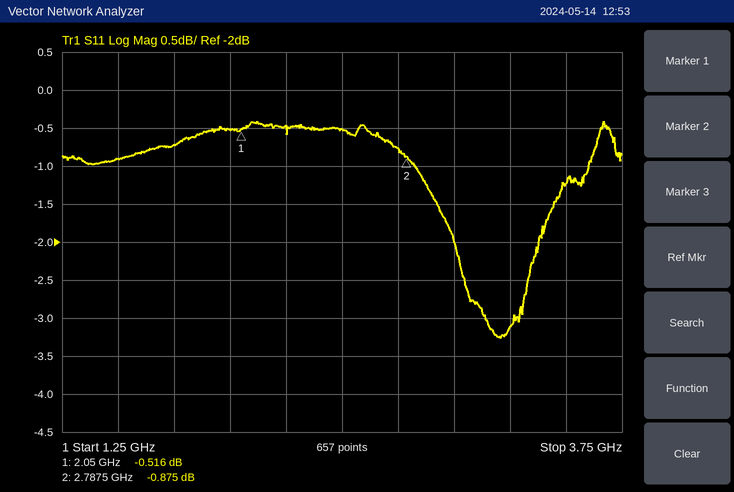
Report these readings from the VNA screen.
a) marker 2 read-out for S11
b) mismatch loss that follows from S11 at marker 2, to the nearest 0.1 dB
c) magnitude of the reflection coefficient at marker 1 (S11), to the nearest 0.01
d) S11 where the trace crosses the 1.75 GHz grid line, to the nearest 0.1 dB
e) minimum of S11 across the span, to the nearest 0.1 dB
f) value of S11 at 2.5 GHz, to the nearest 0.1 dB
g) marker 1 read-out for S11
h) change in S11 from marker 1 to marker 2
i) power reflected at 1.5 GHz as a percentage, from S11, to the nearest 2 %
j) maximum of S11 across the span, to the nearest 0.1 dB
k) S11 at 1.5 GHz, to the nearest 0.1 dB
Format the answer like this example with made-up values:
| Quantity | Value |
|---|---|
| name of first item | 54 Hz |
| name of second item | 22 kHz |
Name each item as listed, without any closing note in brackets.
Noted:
| Quantity | Value |
|---|---|
| marker 2 read-out for S11 | -0.875 dB |
| mismatch loss that follows from S11 at marker 2, to the nearest 0.1 dB | 7.4 dB |
| magnitude of the reflection coefficient at marker 1 (S11), to the nearest 0.01 | 0.94 |
| S11 where the trace crosses the 1.75 GHz grid line, to the nearest 0.1 dB | -0.7 dB |
| minimum of S11 across the span, to the nearest 0.1 dB | -3.3 dB |
| value of S11 at 2.5 GHz, to the nearest 0.1 dB | -0.5 dB |
| marker 1 read-out for S11 | -0.516 dB |
| change in S11 from marker 1 to marker 2 | -0.359 dB |
| power reflected at 1.5 GHz as a percentage, from S11, to the nearest 2 % | 82 % |
| maximum of S11 across the span, to the nearest 0.1 dB | -0.4 dB |
| S11 at 1.5 GHz, to the nearest 0.1 dB | -0.9 dB |
